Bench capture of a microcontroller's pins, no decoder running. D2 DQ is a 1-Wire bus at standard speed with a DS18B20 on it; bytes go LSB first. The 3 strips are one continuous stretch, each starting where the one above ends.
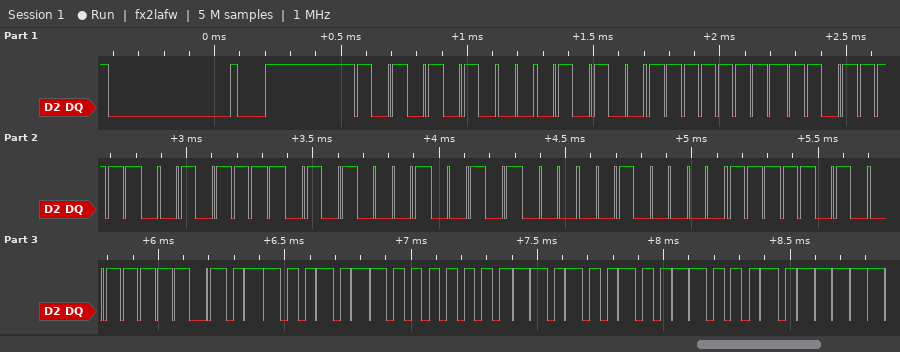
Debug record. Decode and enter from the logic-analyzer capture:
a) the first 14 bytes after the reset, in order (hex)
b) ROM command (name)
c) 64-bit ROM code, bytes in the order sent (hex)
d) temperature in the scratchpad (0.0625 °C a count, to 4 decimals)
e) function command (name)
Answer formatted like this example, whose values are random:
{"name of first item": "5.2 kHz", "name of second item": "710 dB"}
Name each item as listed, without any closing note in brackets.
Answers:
{"the first 14 bytes after the reset, in order": "55 28 FF FB F4 8A 14 04 5F BE A6 01 4B 46", "ROM command": "Match ROM", "64-bit ROM code, bytes in the order sent": "28 FF FB F4 8A 14 04 5F", "temperature in the scratchpad": "26.3750 °C", "function command": "Read Scratchpad"}
